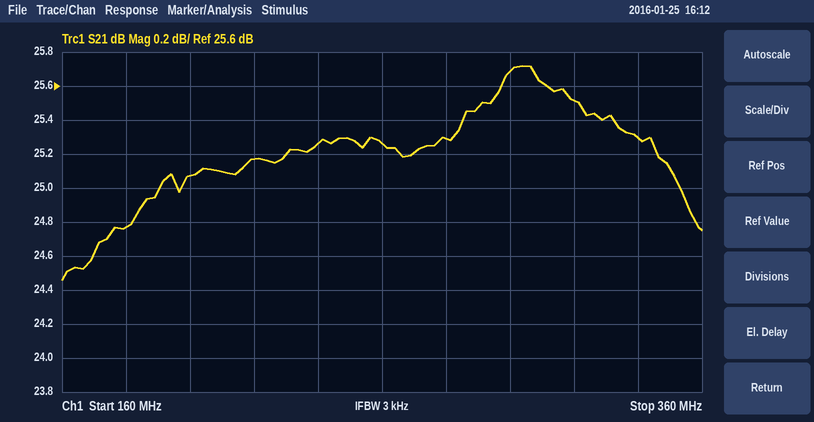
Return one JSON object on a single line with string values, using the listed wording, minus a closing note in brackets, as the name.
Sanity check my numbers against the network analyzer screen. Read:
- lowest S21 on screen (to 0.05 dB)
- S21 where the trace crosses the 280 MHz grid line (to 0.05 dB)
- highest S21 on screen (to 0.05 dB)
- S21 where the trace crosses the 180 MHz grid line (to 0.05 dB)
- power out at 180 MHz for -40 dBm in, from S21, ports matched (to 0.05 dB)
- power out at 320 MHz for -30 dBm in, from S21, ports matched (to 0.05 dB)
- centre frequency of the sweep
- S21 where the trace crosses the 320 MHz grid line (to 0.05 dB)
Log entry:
{"lowest S21 on screen": "24.45 dB", "S21 where the trace crosses the 280 MHz grid line": "25.30 dB", "highest S21 on screen": "25.70 dB", "S21 where the trace crosses the 180 MHz grid line": "24.75 dB", "power out at 180 MHz for -40 dBm in, from S21, ports matched": "-15.25 dBm", "power out at 320 MHz for -30 dBm in, from S21, ports matched": "-4.50 dBm", "centre frequency of the sweep": "260 MHz", "S21 where the trace crosses the 320 MHz grid line": "25.50 dB"}
